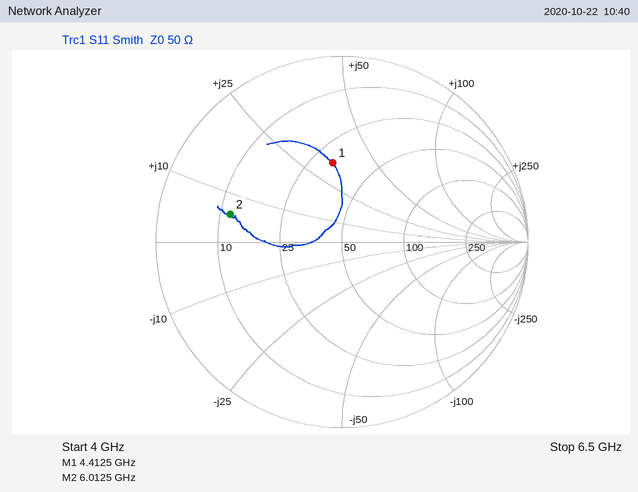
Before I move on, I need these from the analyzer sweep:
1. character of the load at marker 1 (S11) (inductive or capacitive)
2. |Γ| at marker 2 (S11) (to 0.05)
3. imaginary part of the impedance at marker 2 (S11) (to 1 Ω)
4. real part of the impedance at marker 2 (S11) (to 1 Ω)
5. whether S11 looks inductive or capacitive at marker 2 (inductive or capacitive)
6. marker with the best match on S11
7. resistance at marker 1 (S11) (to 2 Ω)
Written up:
inductive
0.60
+6 Ω
12 Ω
inductive
marker 1
32 Ω
